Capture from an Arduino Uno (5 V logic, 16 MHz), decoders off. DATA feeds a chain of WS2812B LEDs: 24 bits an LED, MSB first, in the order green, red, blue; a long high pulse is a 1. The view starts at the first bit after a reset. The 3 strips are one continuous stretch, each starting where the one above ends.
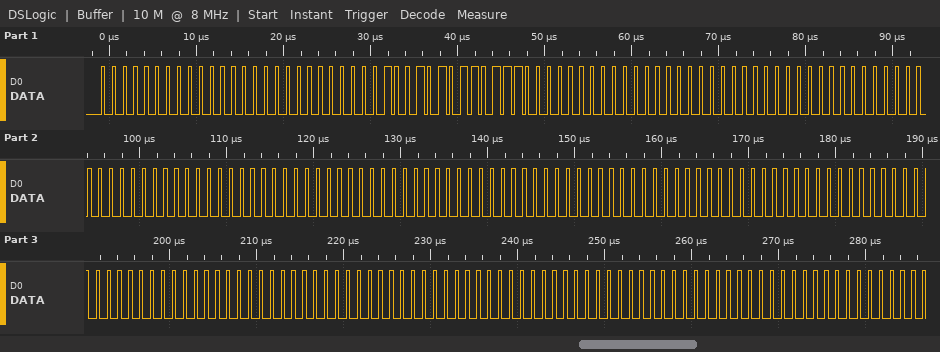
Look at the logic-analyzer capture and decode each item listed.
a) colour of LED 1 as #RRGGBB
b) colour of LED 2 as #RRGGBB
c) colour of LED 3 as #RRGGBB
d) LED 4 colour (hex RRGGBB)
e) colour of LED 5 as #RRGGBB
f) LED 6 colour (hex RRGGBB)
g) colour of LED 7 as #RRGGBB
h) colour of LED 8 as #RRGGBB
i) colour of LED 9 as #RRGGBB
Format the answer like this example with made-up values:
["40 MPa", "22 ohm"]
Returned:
["#000000", "#6E2500", "#000000", "#000000", "#000000", "#000000", "#000000", "#000000", "#000000"]
